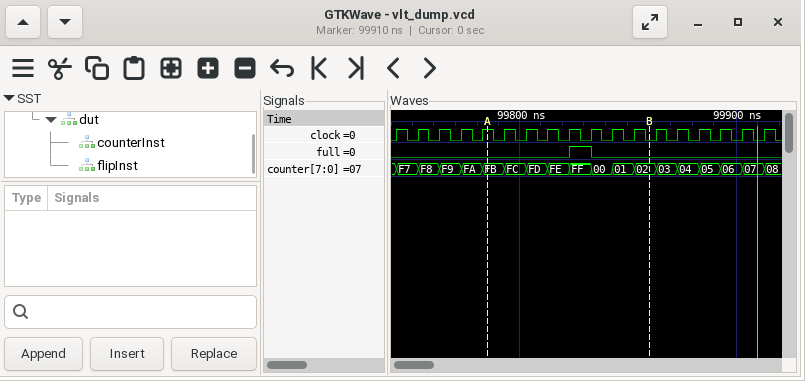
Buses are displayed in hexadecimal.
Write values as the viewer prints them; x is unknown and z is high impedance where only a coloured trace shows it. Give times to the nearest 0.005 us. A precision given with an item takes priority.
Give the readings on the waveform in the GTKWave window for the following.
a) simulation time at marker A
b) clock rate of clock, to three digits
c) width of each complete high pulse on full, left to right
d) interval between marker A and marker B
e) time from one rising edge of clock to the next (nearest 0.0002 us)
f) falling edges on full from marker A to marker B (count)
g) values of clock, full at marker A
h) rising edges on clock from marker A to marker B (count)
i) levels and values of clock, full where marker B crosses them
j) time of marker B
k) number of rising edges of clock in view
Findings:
99.785 us
100 MHz
0.01 us
0.075 us
0.01 us
1
clock=1, full=0
7
clock=0, full=0
99.86 us
18
